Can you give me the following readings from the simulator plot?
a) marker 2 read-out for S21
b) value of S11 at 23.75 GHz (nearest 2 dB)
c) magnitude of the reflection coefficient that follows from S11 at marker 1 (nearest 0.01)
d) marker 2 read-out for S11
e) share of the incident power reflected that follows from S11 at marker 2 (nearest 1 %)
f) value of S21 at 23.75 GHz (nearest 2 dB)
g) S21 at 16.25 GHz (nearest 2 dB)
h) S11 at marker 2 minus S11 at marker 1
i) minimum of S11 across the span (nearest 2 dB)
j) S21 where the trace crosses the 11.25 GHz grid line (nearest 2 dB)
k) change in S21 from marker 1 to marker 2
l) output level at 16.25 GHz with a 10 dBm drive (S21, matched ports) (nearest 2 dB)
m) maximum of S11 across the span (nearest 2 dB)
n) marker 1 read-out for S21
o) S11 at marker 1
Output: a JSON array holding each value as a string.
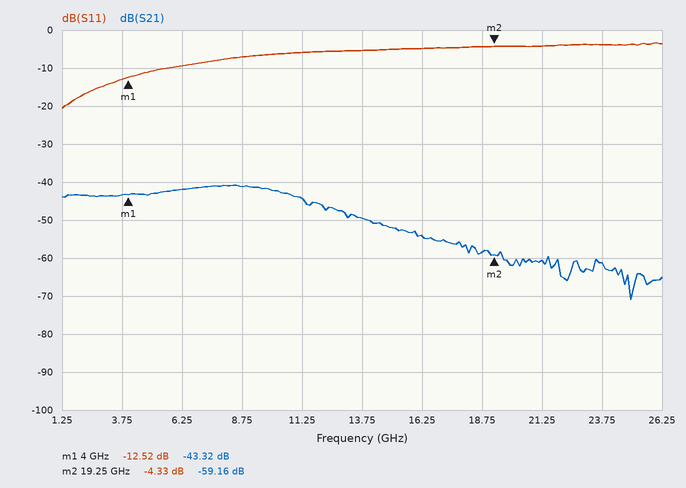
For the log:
["-59.16 dB", "-4 dB", "0.24", "-4.33 dB", "37 %", "-62 dB", "-54 dB", "8.19 dB", "-20 dB", "-44 dB", "-15.84 dB", "-44 dBm", "-4 dB", "-43.32 dB", "-12.52 dB"]
